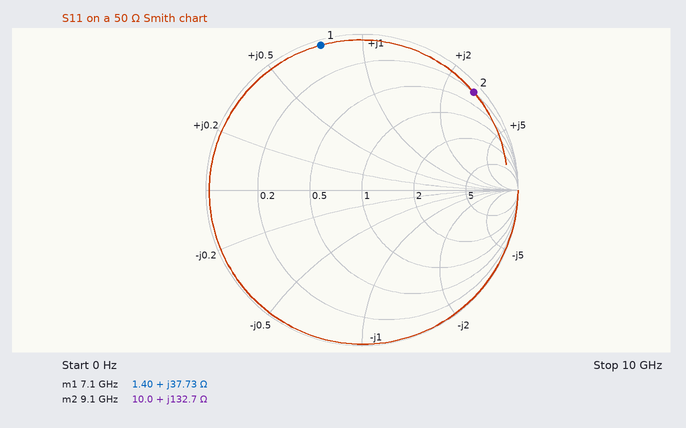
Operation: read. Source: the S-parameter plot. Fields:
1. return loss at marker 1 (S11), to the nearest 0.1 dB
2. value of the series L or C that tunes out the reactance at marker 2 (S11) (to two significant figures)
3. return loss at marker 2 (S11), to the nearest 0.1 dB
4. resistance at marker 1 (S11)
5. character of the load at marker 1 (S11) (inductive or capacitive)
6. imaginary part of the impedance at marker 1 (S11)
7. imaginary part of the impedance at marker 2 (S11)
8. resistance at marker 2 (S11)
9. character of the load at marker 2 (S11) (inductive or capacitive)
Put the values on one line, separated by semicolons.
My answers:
0.3 dB; 130 fF; 0.4 dB; 1.40 Ω; inductive; +37.73 Ω; +132.7 Ω; 10.0 Ω; inductive
